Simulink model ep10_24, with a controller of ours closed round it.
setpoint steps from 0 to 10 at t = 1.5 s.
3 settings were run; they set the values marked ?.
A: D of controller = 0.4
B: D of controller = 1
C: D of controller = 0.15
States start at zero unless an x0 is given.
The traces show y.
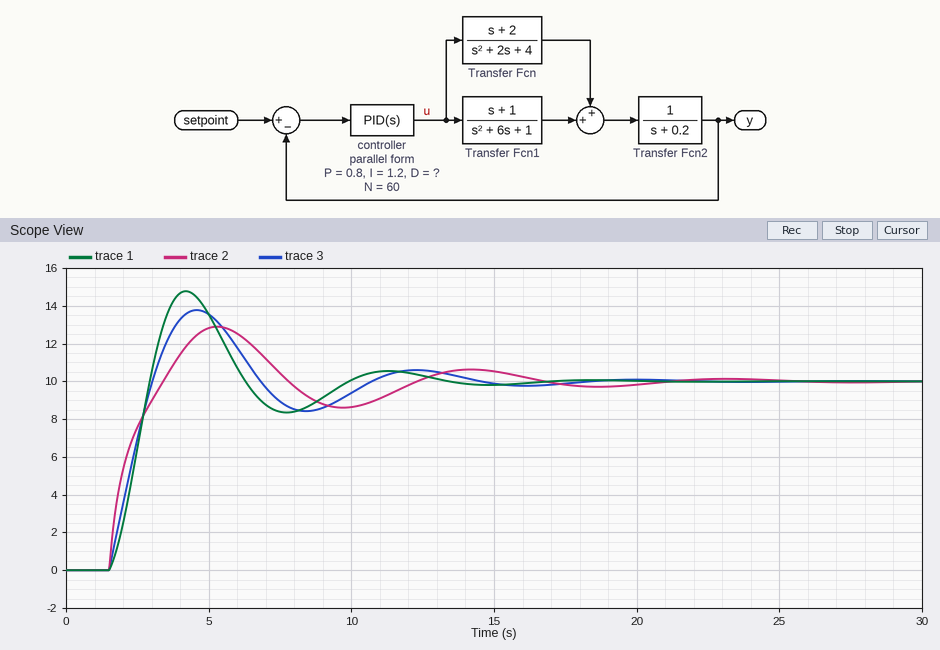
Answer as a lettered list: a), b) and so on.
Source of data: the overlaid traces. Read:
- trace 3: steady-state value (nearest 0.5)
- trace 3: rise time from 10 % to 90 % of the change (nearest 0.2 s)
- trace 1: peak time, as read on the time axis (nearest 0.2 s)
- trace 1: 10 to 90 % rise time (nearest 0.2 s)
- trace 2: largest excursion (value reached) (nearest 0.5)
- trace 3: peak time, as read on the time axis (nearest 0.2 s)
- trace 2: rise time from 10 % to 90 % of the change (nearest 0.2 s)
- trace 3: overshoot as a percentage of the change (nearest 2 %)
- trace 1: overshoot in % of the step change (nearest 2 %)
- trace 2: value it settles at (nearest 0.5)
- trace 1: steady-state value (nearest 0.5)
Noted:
a) 10.0
b) 1.2 s
c) 4.2 s
d) 1.0 s
e) 13.0
f) 4.6 s
g) 1.4 s
h) 38 %
i) 48 %
j) 10.0
k) 10.0
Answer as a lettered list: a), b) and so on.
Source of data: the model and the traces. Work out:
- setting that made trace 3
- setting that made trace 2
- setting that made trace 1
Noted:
a) A
b) B
c) C
